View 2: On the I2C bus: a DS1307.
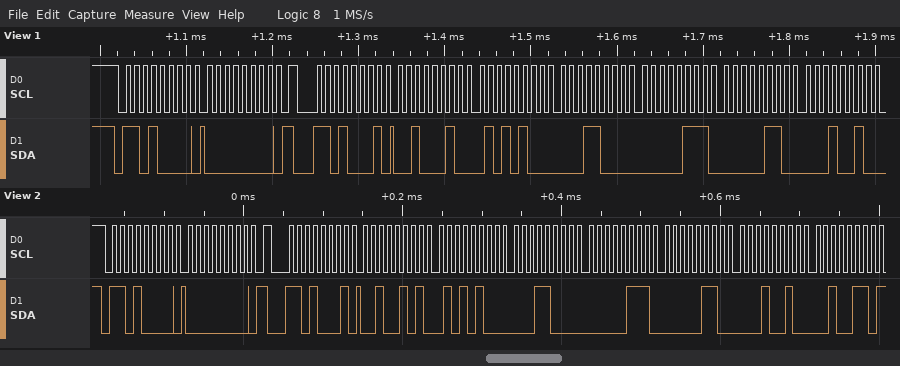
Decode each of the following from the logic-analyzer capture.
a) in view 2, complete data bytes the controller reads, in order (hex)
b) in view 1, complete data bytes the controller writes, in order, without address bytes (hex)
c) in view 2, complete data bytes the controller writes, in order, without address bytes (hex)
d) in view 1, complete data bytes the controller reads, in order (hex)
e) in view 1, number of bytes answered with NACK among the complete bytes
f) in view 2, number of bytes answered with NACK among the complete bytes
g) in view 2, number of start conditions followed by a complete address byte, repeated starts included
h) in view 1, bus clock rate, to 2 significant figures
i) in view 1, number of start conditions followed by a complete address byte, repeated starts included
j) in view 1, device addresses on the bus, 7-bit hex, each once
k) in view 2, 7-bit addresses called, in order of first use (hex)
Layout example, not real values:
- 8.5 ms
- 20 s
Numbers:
- 25 54 18 07 06 12 26
- 00
- 00
- 22 54 18 07 06 12
- 0
- 1
- 2
- 100 kHz
- 2
- 0x68
- 0x68
